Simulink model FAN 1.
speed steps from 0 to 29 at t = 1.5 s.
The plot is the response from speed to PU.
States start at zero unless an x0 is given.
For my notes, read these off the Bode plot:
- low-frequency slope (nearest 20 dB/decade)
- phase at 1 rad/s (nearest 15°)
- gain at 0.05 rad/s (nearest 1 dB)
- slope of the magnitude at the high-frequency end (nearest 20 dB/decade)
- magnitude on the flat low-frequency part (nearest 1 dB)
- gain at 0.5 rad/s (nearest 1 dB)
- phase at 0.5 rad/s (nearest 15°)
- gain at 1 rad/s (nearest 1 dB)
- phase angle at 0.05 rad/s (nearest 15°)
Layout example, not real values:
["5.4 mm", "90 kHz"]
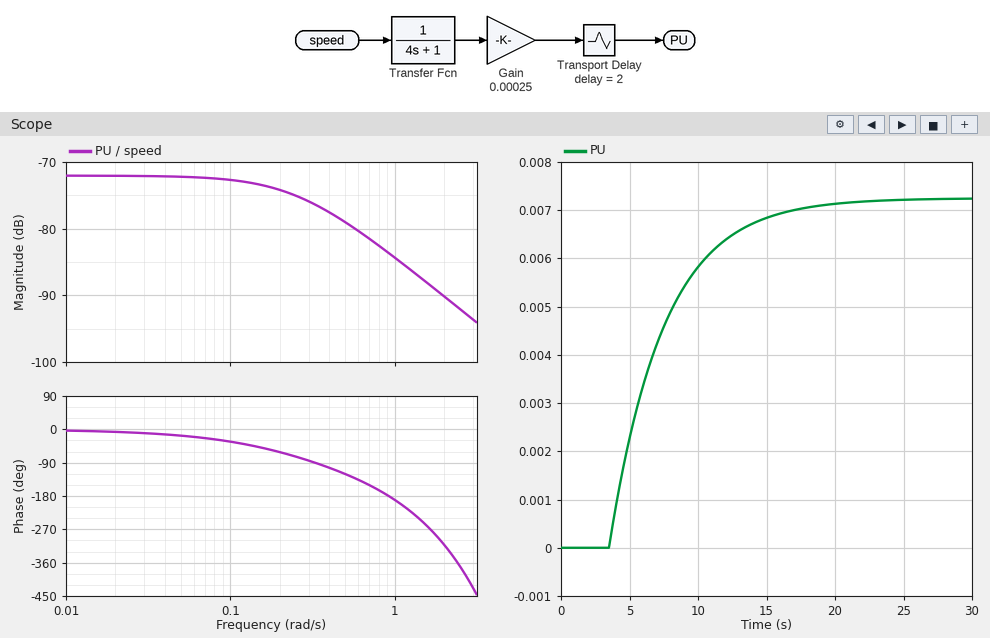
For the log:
["0 dB/decade", "-195°", "-72 dB", "-20 dB/decade", "-72 dB", "-79 dB", "-120°", "-84 dB", "-15°"]
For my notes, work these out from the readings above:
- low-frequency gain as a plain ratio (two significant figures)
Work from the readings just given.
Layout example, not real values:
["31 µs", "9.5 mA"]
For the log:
["0.00025"]
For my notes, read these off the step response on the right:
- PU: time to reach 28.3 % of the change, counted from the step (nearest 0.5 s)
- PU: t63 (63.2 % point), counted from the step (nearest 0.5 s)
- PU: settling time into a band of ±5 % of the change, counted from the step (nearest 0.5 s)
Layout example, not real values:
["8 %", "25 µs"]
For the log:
["3.5 s", "6.0 s", "14.0 s"]
